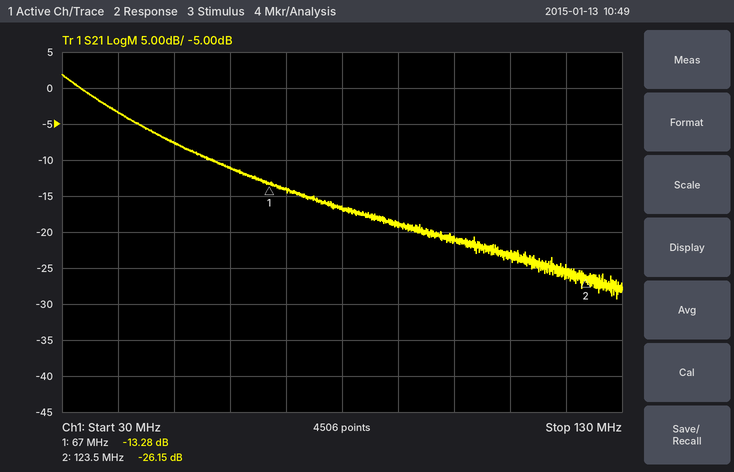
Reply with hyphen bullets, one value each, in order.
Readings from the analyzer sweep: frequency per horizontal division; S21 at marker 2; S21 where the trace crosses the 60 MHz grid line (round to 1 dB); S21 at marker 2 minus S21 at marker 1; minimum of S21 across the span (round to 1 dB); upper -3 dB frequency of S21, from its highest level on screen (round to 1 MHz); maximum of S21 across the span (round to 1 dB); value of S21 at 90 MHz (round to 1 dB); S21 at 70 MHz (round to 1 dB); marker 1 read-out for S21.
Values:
- 10 MHz
- -26.15 dB
- -11 dB
- -12.87 dB
- -29 dB
- 35 MHz
- 2 dB
- -19 dB
- -14 dB
- -13.28 dB
